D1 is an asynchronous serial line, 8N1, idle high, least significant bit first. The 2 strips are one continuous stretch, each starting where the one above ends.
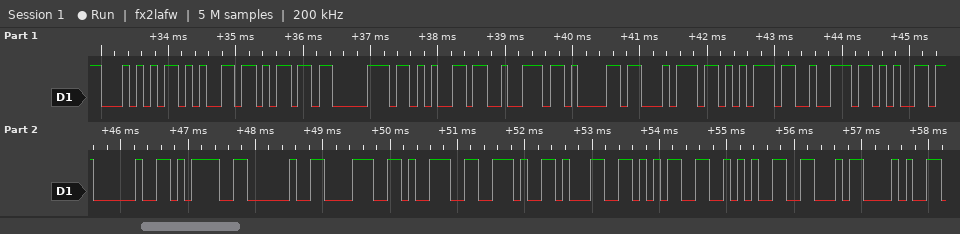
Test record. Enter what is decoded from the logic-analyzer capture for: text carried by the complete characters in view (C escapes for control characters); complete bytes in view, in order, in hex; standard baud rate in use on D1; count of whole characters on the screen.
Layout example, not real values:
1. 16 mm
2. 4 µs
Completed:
1. "Temperature = 89.15*F("
2. 54 65 6D 70 65 72 61 74 75 72 65 20 3D 20 38 39 2E 31 35 2A 46 28
3. 9600 baud
4. 22
